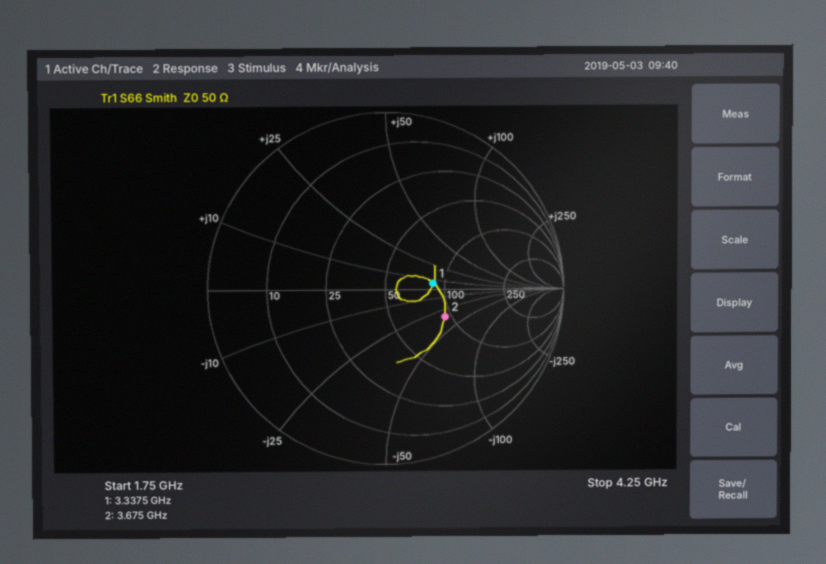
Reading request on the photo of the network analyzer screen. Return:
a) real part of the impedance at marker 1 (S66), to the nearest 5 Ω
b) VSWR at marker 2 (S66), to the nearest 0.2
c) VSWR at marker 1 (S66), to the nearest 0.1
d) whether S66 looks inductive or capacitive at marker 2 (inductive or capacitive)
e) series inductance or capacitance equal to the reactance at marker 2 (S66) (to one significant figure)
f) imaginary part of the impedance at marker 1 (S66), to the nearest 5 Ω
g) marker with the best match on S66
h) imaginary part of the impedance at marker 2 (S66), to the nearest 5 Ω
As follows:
85 Ω
2.2
1.7
capacitive
1 pF
+5 Ω
marker 1
-35 Ω
